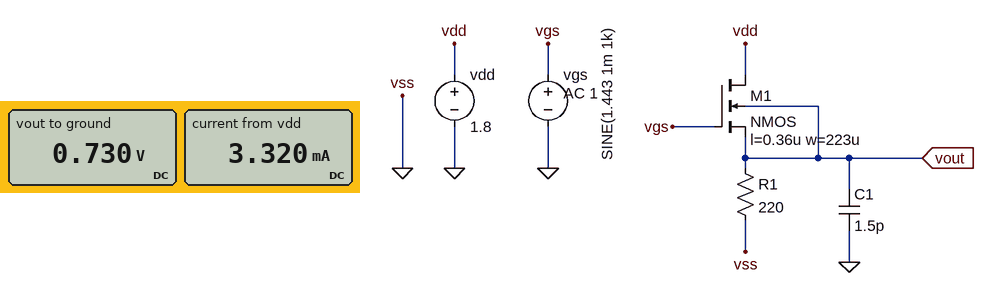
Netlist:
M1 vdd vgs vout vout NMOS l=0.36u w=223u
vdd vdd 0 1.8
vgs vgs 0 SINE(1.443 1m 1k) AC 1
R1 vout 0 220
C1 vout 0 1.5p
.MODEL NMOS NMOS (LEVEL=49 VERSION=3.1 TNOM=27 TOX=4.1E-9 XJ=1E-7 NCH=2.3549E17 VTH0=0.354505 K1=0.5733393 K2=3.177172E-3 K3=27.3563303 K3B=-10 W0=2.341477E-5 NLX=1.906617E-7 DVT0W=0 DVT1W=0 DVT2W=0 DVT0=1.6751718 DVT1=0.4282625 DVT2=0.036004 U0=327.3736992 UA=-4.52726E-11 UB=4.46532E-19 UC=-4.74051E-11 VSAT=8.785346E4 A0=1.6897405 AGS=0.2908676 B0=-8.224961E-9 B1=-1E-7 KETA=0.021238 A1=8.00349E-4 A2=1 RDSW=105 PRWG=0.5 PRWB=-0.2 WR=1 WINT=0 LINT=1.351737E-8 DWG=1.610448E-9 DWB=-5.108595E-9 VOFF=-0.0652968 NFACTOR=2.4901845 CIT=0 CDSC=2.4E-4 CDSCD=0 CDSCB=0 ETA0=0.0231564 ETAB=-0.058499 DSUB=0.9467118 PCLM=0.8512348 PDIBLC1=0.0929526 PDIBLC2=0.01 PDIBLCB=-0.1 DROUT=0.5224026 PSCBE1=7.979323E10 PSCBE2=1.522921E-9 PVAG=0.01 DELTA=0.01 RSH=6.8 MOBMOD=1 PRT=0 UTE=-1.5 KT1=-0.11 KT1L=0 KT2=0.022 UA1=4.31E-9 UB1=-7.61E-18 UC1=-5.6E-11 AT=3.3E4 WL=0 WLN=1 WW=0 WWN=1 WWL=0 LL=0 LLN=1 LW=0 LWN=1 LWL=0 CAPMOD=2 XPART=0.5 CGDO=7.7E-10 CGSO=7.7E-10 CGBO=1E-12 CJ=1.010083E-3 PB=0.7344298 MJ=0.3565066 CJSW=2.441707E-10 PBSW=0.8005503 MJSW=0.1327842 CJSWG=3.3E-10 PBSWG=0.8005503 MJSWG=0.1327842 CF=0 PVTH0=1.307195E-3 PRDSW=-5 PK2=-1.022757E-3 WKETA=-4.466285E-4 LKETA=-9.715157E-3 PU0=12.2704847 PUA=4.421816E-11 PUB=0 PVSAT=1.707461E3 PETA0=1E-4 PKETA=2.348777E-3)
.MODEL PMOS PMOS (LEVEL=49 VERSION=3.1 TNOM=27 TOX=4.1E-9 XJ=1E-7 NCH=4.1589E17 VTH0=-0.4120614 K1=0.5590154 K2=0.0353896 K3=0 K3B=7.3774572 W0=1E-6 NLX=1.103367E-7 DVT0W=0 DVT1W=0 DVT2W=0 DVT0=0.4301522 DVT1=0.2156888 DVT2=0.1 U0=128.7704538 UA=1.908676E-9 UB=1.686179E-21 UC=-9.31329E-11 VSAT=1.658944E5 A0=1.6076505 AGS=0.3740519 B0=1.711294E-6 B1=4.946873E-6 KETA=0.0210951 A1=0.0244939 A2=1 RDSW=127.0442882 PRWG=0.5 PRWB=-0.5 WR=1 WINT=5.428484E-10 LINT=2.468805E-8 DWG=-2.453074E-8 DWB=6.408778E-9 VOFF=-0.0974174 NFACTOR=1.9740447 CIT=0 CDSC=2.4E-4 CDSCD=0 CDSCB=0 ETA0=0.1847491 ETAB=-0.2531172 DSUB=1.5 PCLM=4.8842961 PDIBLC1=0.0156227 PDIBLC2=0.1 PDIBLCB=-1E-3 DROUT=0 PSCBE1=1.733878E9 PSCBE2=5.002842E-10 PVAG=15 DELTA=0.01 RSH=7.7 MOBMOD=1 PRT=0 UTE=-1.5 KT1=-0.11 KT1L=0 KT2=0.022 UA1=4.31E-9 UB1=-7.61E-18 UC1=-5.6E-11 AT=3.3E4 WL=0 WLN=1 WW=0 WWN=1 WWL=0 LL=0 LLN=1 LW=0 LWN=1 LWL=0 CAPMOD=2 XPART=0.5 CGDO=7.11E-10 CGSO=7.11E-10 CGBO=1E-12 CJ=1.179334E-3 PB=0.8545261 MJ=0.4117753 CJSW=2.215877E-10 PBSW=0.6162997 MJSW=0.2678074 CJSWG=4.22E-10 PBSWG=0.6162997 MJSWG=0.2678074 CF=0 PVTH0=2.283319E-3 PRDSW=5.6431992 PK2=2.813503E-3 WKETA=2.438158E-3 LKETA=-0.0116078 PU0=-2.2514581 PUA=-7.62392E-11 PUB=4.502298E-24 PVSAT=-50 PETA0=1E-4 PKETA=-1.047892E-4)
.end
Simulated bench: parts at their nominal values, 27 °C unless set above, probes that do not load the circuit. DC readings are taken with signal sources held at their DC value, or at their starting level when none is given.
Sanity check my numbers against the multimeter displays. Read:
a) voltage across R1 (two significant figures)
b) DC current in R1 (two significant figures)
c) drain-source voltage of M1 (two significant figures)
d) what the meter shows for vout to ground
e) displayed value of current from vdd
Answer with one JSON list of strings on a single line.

["730 mV", "3.3 mA", "1.1 V", "0.730 V", "3.320 mA"]
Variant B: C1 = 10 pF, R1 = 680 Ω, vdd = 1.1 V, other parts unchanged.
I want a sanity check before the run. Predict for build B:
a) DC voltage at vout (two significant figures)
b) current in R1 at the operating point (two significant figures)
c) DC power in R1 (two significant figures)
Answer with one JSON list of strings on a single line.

["820 mV", "1.2 mA", "990 µW"]
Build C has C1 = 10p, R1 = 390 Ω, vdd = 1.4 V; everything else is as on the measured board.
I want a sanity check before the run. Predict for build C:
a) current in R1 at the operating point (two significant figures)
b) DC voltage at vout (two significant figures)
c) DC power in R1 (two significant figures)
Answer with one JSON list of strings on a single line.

["2.0 mA", "780 mV", "1.6 mW"]
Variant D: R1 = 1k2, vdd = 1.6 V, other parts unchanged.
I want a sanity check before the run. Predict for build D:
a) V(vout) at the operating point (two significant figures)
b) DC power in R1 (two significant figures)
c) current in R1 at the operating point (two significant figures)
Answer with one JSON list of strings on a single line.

["860 mV", "620 µW", "720 µA"]
